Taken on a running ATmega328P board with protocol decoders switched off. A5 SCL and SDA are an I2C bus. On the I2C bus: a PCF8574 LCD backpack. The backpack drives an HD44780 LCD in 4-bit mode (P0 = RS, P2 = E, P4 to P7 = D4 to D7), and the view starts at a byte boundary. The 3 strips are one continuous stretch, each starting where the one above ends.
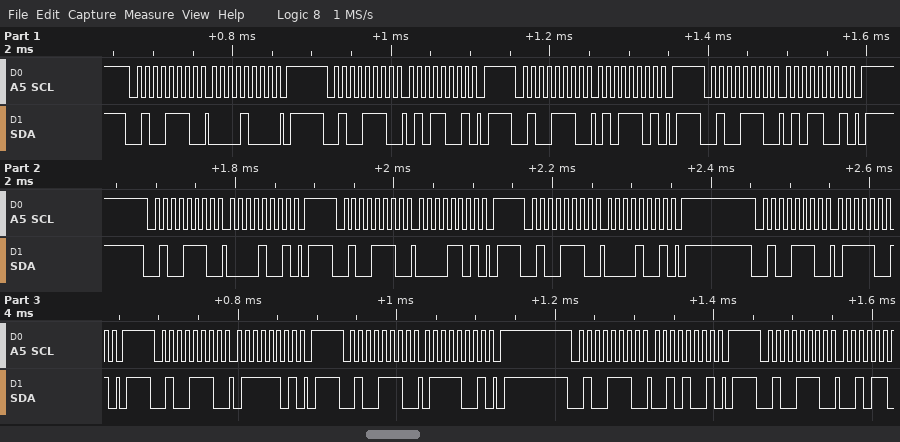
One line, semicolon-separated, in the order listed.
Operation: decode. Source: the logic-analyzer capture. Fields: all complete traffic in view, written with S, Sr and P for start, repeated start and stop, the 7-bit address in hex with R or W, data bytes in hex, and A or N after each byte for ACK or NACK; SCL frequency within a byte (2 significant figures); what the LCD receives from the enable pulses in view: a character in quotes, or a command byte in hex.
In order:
S 27W A 08 A P S 27W A 59 A P S 27W A 5D A P S 27W A 59 A P S 27W A 09 A P S 27W A 0D A P S 27W A 09 A P S 27W A 79 A P S 27W A 7D A P S 27W A 79 A P S 27W A 29 A P S 27W A; 100 kHz; 'P'
